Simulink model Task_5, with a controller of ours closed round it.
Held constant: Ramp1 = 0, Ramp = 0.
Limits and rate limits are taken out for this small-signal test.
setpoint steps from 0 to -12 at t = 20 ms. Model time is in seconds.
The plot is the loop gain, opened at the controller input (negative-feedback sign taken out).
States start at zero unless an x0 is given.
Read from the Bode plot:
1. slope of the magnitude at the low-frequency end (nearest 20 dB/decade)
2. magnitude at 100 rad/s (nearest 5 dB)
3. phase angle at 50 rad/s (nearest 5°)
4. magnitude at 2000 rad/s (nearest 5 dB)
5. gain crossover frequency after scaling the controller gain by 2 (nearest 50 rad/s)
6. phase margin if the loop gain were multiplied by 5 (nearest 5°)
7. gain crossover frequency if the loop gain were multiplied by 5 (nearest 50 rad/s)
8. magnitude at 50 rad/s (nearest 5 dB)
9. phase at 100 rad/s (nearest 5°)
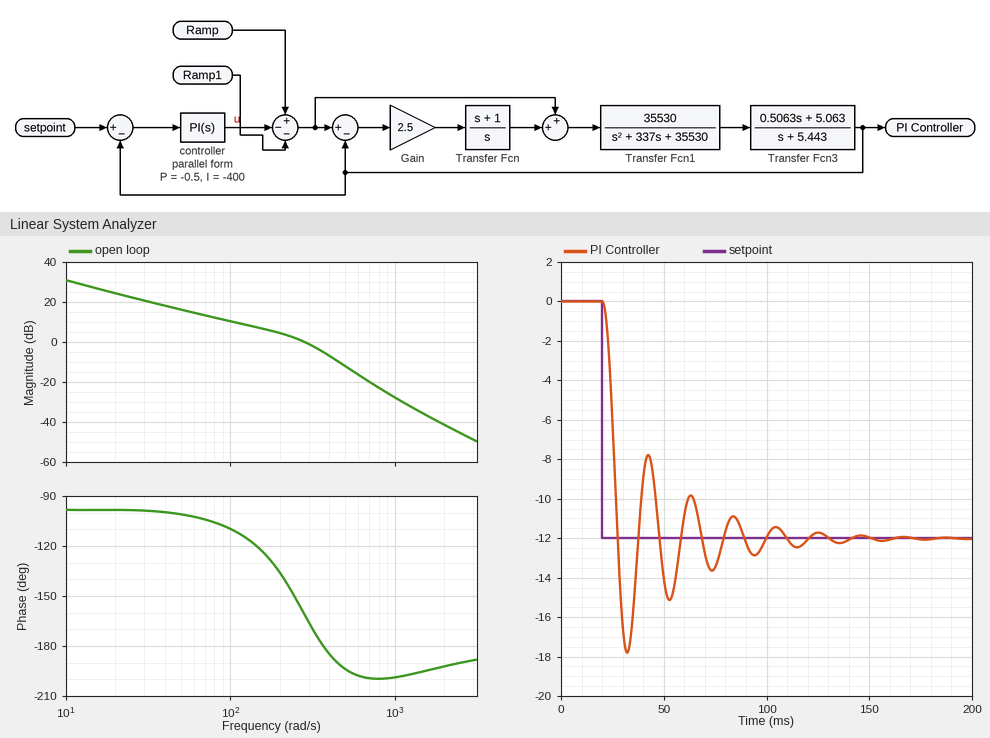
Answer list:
-20 dB/decade
10 dB
-100°
-40 dB
400 rad/s
-15°
550 rad/s
15 dB
-110°
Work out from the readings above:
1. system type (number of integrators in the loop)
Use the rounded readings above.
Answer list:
1
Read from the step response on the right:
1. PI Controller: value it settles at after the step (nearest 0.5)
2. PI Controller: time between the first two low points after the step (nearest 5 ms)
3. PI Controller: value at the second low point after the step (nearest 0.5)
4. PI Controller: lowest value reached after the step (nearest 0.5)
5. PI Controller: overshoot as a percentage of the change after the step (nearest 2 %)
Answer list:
-12.0
20 ms
-15.0
-18.0
48 %
